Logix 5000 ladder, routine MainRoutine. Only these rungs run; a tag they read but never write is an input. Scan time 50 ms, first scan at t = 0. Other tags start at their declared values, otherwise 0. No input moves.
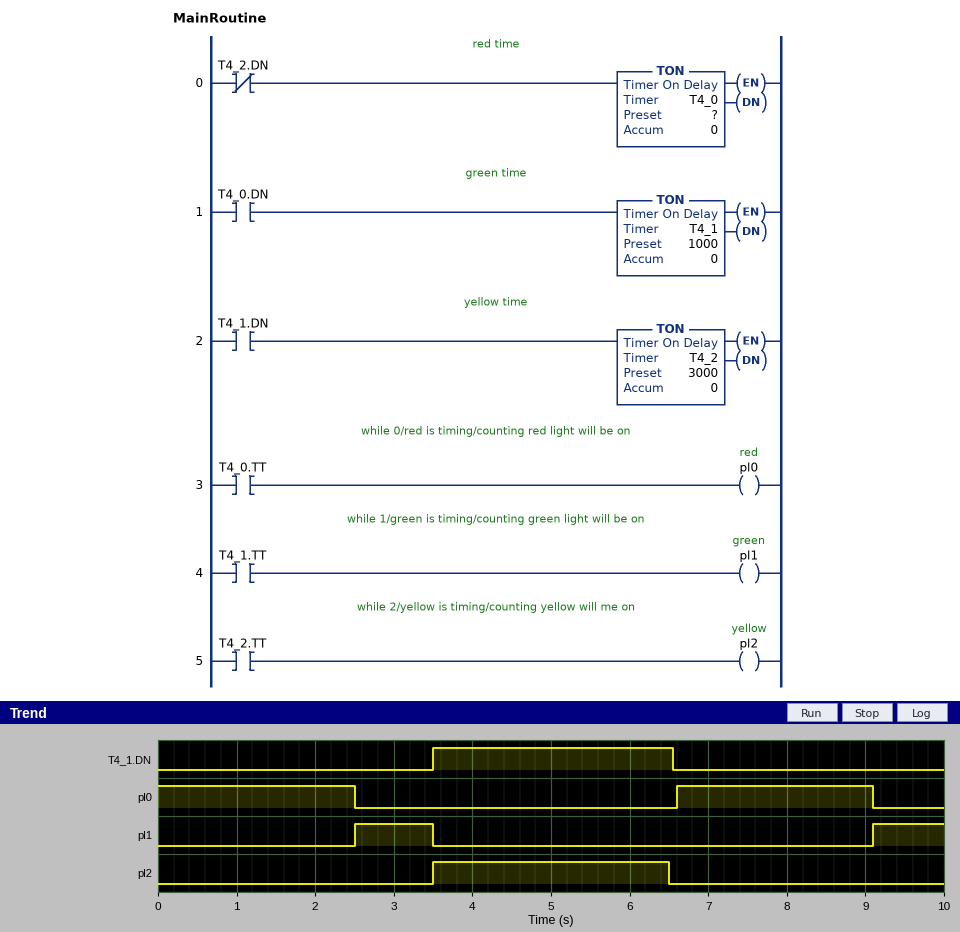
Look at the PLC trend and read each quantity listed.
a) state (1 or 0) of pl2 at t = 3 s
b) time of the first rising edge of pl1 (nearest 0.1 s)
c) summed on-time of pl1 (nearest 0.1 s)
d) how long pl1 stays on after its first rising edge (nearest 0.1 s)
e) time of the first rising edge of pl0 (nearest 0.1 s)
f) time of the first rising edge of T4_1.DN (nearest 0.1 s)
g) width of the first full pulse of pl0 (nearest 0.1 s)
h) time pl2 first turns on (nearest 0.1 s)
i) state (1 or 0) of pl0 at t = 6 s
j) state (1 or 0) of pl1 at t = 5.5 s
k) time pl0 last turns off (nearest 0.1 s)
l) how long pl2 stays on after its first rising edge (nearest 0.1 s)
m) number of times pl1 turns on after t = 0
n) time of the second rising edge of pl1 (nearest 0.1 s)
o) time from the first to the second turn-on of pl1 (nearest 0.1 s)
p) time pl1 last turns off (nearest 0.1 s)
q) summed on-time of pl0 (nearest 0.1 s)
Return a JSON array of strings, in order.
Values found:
["0", "2.5 s", "1.9 s", "1.0 s", "6.6 s", "3.5 s", "2.5 s", "3.5 s", "0", "0", "9.1 s", "3.0 s", "2", "9.1 s", "6.6 s", "3.5 s", "5.0 s"]
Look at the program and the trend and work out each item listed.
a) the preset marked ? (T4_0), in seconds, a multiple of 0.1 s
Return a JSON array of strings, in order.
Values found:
["2.5 s"]
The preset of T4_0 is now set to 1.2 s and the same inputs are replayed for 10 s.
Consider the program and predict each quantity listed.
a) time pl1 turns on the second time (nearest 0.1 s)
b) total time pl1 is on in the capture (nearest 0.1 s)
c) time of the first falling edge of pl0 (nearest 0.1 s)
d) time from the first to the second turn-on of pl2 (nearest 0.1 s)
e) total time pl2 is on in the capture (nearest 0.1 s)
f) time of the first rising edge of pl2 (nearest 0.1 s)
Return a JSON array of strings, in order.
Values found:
["6.5 s", "2.0 s", "1.2 s", "5.3 s", "5.5 s", "2.2 s"]
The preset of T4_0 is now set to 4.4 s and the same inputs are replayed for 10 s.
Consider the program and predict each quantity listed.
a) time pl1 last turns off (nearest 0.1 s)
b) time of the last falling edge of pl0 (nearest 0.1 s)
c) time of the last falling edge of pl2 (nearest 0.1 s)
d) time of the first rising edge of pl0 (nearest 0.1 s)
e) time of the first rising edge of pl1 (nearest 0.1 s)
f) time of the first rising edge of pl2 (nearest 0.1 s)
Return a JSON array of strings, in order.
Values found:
["5.4 s", "4.4 s", "8.4 s", "8.5 s", "4.4 s", "5.4 s"]
